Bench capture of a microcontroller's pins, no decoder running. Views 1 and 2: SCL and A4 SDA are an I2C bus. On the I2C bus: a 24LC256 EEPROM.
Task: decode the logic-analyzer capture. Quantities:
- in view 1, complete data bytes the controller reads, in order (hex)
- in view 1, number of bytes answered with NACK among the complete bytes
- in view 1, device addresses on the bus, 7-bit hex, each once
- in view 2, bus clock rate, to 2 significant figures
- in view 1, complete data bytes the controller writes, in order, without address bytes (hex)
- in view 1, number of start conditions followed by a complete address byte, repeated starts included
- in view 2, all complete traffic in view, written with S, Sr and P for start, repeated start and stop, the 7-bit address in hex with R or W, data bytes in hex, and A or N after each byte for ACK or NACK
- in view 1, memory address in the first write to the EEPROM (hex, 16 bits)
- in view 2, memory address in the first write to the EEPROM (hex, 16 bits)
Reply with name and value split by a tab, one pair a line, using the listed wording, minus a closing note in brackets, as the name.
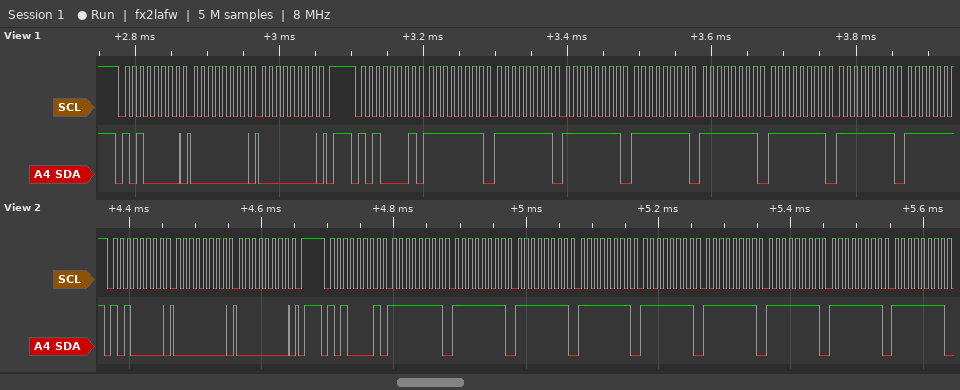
in view 1, complete data bytes the controller reads, in order	FF FF FF FF FF FF FF
in view 1, number of bytes answered with NACK among the complete bytes	0
in view 1, device addresses on the bus, 7-bit hex, each once	0x50
in view 2, bus clock rate, to 2 significant figures	100 kHz
in view 1, complete data bytes the controller writes, in order, without address bytes	00 00
in view 1, number of start conditions followed by a complete address byte, repeated starts included	2
in view 2, all complete traffic in view, written with S, Sr and P for start, repeated start and stop, the 7-bit address in hex with R or W, data bytes in hex, and A or N after each byte for ACK or NACK	S 50W A 00 A 00 A P S 50R A FF A FF A FF A FF A FF A FF A FF A FF A FF A
in view 1, memory address in the first write to the EEPROM	0x0000
in view 2, memory address in the first write to the EEPROM	0x0000
